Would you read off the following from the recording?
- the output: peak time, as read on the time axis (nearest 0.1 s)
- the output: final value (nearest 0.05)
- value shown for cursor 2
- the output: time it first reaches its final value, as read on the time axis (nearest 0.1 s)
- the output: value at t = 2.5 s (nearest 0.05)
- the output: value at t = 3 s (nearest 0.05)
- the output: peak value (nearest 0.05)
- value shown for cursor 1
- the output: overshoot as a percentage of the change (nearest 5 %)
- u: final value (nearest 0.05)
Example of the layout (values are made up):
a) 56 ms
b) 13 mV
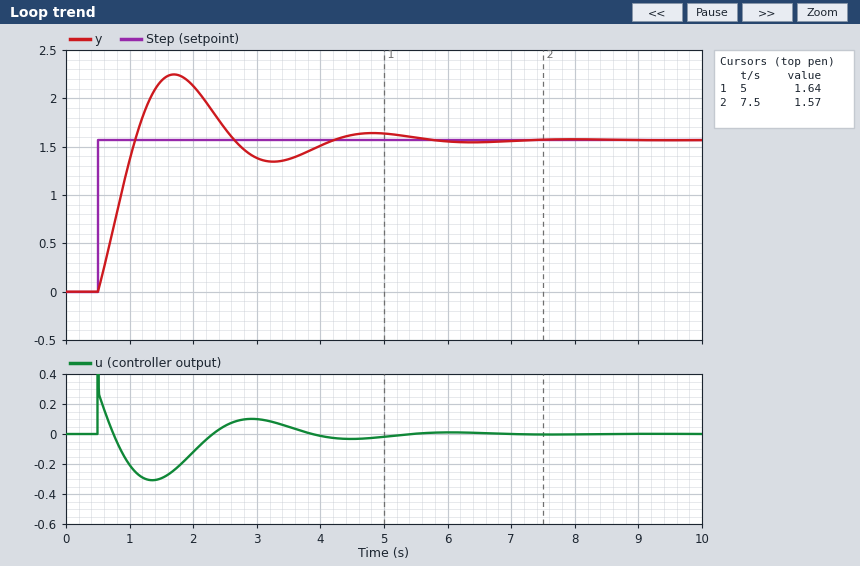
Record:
a) 1.7 s
b) 1.55
c) 1.57
d) 1.1 s
e) 1.70
f) 1.40
g) 2.25
h) 1.64
i) 45 %
j) 0.00
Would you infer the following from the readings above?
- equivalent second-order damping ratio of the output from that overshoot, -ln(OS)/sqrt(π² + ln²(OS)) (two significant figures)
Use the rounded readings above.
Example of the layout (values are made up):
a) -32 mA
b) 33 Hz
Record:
a) 0.25
